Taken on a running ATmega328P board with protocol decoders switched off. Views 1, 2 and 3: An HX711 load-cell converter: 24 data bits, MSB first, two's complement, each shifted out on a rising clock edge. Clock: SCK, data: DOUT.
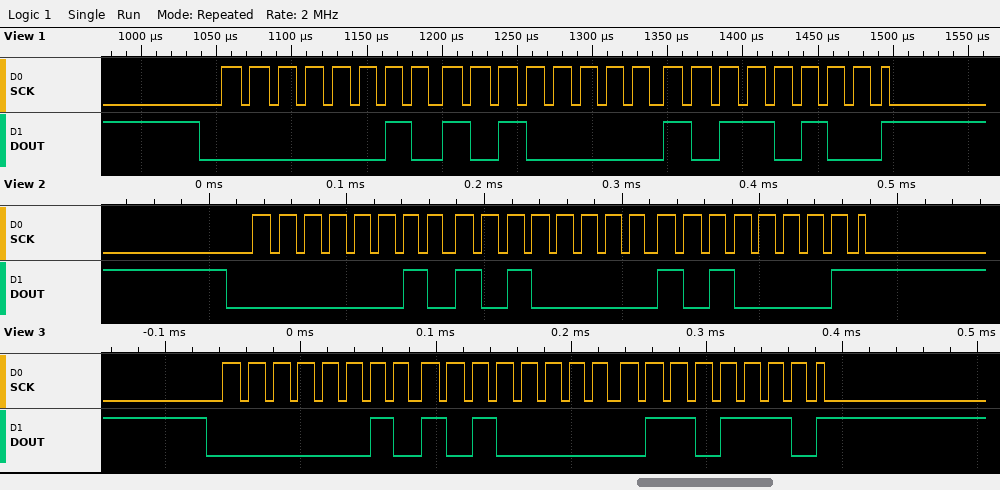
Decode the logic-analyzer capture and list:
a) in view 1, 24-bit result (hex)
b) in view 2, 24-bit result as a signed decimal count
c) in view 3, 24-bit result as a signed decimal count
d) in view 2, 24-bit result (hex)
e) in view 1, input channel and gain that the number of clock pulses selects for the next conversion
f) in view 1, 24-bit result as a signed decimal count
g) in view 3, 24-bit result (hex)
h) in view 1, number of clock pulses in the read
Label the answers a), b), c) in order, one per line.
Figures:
a) 0x02A0B4
b) 172193
c) 172142
d) 0x02A0A1
e) channel A, gain 128
f) 172212
g) 0x02A06E
h) 25
